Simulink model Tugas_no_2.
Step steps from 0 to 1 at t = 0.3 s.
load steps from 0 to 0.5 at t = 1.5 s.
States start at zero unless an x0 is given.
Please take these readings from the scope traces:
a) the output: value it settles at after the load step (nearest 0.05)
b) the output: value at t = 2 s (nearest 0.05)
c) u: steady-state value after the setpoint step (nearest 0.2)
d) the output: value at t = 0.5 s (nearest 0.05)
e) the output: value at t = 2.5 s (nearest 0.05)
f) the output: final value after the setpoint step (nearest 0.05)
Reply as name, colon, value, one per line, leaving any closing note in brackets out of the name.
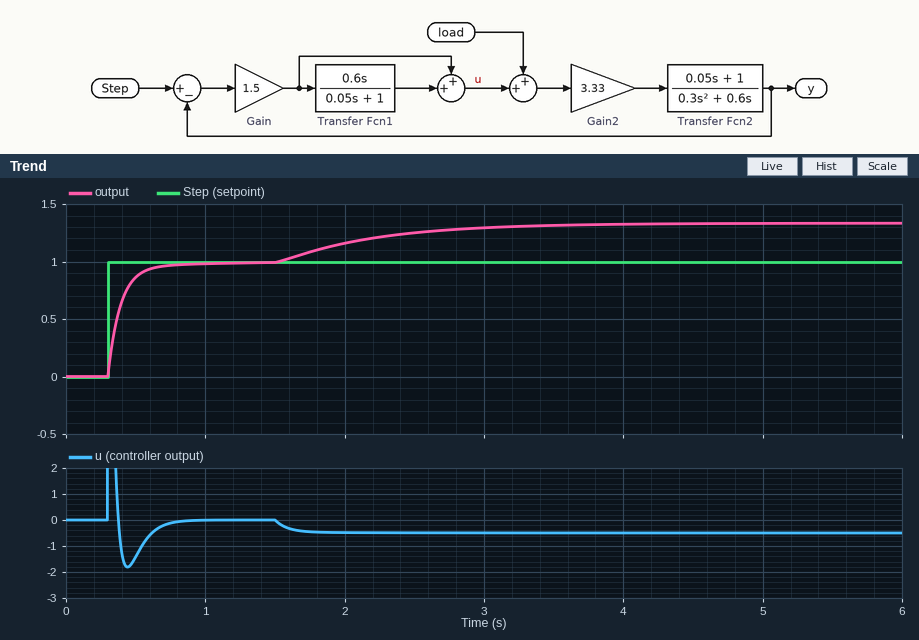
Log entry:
the output: value it settles at after the load step: 1.35
the output: value at t = 2 s: 1.15
u: steady-state value after the setpoint step: 0.0
the output: value at t = 0.5 s: 0.85
the output: value at t = 2.5 s: 1.25
the output: final value after the setpoint step: 1.00
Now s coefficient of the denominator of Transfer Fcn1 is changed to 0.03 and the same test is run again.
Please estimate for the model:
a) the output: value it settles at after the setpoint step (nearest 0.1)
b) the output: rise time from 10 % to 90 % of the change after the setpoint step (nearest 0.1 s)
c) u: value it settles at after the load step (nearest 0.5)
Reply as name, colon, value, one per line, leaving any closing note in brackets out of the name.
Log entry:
the output: value it settles at after the setpoint step: 1.0
the output: rise time from 10 % to 90 % of the change after the setpoint step: 0.3 s
u: value it settles at after the load step: -0.5
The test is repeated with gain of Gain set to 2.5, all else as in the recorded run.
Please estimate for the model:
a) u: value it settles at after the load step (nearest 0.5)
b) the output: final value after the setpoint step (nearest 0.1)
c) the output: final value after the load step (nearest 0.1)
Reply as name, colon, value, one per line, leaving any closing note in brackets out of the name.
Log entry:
u: value it settles at after the load step: -0.5
the output: final value after the setpoint step: 1.0
the output: final value after the load step: 1.2
